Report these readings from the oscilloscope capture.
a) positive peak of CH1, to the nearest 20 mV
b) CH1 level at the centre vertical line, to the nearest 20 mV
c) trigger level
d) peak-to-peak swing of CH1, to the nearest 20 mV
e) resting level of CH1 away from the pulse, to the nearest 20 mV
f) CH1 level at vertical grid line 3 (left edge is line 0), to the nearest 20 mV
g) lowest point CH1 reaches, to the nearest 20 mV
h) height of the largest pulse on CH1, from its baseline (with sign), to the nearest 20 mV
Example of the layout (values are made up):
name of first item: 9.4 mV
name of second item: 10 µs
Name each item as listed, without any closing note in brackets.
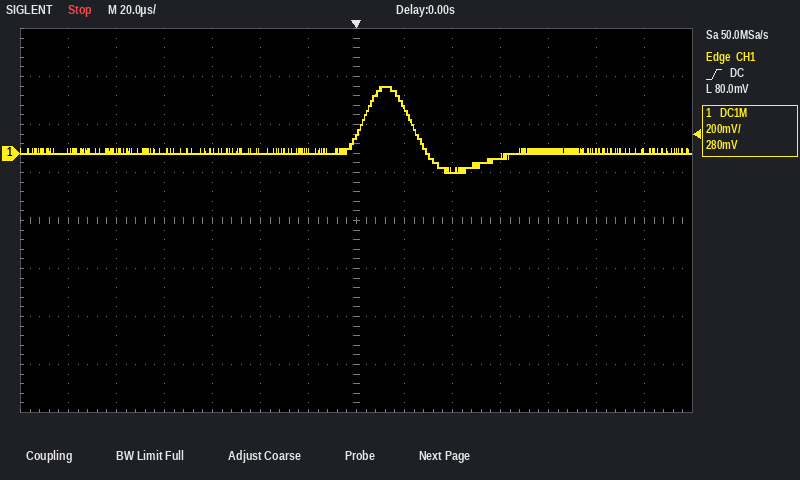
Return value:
positive peak of CH1, to the nearest 20 mV: 280 mV
CH1 level at the centre vertical line, to the nearest 20 mV: 80 mV
trigger level: 80.0 mV
peak-to-peak swing of CH1, to the nearest 20 mV: 360 mV
resting level of CH1 away from the pulse, to the nearest 20 mV: 0 mV
CH1 level at vertical grid line 3 (left edge is line 0), to the nearest 20 mV: 0 mV
lowest point CH1 reaches, to the nearest 20 mV: -80 mV
height of the largest pulse on CH1, from its baseline (with sign), to the nearest 20 mV: +280 mV
